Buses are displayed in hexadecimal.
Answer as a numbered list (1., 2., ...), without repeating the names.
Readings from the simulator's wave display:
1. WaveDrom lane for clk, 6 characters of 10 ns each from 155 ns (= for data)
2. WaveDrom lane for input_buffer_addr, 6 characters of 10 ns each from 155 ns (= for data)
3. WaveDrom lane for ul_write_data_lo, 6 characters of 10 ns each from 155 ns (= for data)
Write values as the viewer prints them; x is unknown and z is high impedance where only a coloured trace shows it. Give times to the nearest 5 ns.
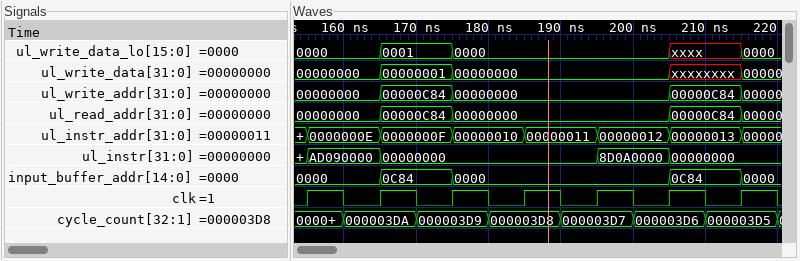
1. {name: 'clk', wave: 'p.....'}
2. {name: 'input_buffer_addr', wave: '===..=', data: '0000 0C84 0000 0C84'}
3. {name: 'ul_write_data_lo', wave: '===..x', data: '0000 0001 0000'}
